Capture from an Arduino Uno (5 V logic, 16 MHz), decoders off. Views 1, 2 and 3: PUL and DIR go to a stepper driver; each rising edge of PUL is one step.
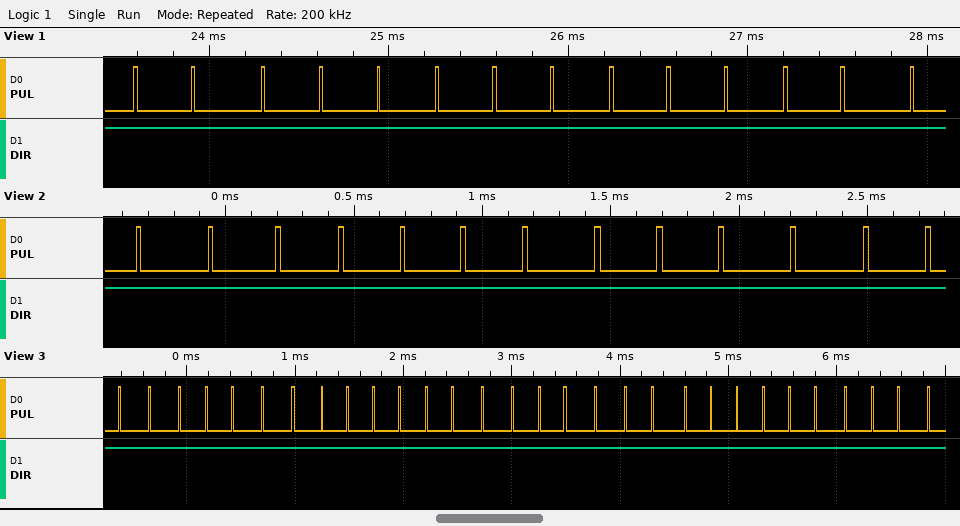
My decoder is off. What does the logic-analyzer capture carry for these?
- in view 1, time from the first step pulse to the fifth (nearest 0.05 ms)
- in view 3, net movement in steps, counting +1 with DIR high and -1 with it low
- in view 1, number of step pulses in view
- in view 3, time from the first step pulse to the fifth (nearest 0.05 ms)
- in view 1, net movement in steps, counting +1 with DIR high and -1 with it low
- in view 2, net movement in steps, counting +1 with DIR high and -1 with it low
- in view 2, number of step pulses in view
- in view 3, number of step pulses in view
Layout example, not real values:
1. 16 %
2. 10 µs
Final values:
1. 1.35 ms
2. +30
3. 14
4. 1.05 ms
5. +14
6. +13
7. 13
8. 30
